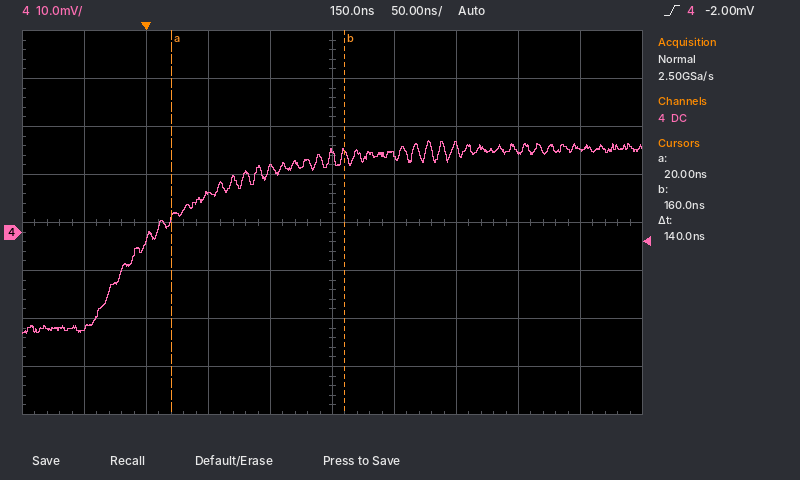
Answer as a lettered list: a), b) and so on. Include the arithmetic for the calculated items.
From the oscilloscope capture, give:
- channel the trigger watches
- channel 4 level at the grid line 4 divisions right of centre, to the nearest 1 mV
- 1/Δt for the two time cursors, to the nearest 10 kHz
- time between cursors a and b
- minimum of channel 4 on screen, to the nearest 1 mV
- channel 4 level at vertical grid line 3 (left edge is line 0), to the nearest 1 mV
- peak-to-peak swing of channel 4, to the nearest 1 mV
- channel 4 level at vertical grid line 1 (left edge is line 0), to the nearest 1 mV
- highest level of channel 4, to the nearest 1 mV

a) channel 4
b) 17 mV
c) 1 / 140 ns ≈ 7.14 MHz
d) 140 ns
e) -21 mV
f) 8 mV
g) 19 mV − (-21 mV) = 40 mV
h) -20 mV
i) 19 mV
